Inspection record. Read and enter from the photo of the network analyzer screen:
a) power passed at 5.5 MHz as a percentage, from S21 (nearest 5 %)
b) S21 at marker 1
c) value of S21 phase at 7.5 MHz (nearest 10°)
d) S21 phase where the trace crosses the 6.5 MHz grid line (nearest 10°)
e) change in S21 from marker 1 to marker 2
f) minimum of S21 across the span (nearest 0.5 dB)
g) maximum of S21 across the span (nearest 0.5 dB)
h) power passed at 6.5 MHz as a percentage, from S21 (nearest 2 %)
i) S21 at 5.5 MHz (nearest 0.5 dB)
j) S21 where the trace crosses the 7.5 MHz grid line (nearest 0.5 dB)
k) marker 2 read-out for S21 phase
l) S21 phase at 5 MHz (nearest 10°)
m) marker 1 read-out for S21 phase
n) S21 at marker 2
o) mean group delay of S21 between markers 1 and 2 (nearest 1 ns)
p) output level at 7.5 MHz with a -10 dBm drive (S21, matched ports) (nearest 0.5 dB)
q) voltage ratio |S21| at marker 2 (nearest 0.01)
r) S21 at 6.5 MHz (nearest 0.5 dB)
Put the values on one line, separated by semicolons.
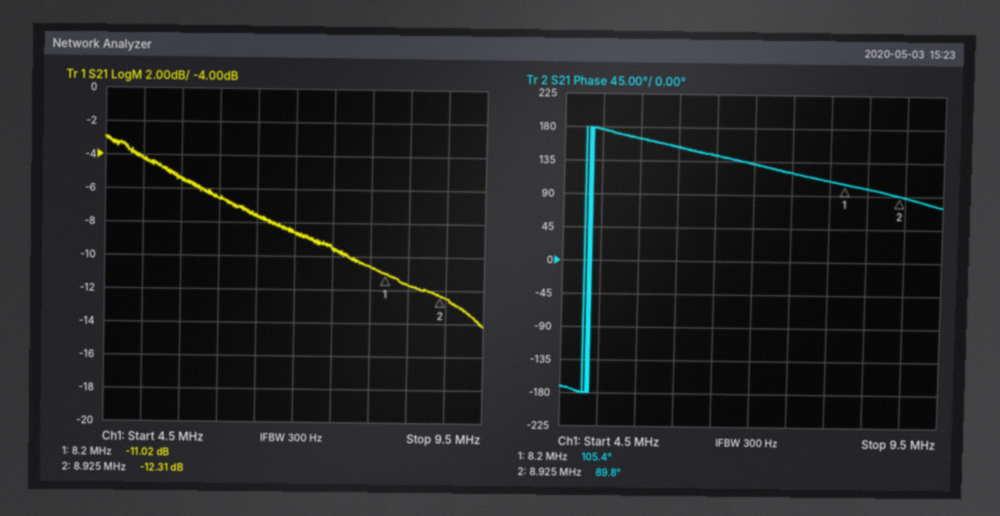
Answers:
30 %; -11.02 dB; 120°; 140°; -1.29 dB; -14.0 dB; -3.0 dB; 18 %; -5.5 dB; -9.5 dB; 89.8°; 180°; 105.4°; -12.31 dB; 60 ns; -19.5 dBm; 0.24; -7.5 dB
